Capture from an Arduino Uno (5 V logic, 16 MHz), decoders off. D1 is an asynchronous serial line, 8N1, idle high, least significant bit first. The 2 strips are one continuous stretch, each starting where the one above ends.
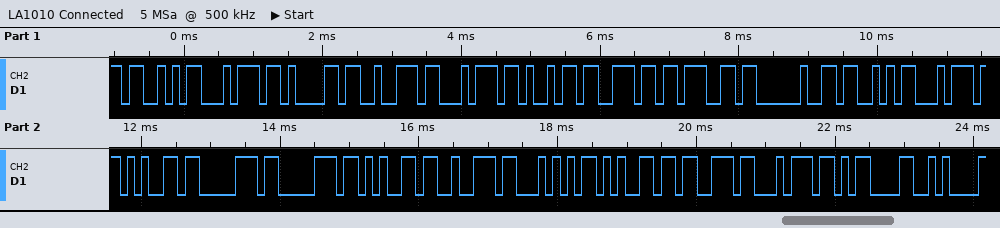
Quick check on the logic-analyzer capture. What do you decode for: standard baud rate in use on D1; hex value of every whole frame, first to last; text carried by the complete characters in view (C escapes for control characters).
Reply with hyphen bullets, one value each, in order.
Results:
- 9600 baud
- 0x53 0x74 0x61 0x72 0x74 0x69 0x6E 0x67 0x20 0x53 0x74 0x65 0x70 0x70 0x65 0x72 0x54 0x65 0x73 0x74 0x0D 0x0A
- "Starting StepperTest\r\n"
